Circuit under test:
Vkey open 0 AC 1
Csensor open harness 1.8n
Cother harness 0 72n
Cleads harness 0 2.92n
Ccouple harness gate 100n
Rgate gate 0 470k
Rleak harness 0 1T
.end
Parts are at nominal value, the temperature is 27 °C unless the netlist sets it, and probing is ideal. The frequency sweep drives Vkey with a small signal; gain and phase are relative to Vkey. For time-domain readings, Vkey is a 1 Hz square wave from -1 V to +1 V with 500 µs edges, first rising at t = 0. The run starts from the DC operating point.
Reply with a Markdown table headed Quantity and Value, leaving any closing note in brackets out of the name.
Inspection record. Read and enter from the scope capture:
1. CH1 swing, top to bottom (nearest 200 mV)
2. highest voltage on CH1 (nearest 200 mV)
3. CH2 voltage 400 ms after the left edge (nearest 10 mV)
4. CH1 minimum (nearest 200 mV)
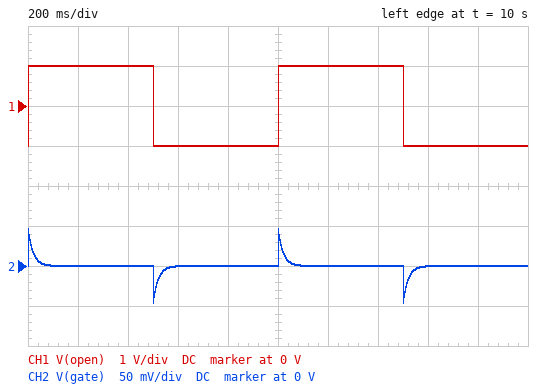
| Quantity | Value |
|---|---|
| CH1 swing, top to bottom | 2.0 V |
| highest voltage on CH1 | 1.0 V |
| CH2 voltage 400 ms after the left edge | 0 V |
| CH1 minimum | -1.0 V |
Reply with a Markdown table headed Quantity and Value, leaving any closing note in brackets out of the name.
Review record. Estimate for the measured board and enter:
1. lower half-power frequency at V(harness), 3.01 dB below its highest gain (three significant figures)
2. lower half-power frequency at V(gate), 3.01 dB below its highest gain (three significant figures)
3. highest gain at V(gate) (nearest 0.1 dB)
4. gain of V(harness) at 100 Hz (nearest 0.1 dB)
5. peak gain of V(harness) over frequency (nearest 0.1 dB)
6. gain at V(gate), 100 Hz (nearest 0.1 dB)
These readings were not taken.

| Quantity | Value |
|---|---|
| lower half-power frequency at V(harness), 3.01 dB below its highest gain | 6.16 Hz |
| lower half-power frequency at V(gate), 3.01 dB below its highest gain | 7.80 Hz |
| highest gain at V(gate) | -32.6 dB |
| gain of V(harness) at 100 Hz | -32.6 dB |
| peak gain of V(harness) over frequency | -32.6 dB |
| gain at V(gate), 100 Hz | -32.6 dB |
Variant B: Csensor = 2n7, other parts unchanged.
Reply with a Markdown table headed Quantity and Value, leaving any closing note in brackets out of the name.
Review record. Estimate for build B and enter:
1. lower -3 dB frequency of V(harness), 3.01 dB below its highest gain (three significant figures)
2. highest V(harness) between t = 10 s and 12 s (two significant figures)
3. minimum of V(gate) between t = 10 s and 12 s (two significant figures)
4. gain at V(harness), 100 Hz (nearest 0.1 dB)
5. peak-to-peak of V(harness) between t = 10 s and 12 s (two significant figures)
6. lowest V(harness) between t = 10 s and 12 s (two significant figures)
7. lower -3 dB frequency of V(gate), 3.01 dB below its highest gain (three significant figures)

| Quantity | Value |
|---|---|
| lower -3 dB frequency of V(harness), 3.01 dB below its highest gain | 6.09 Hz |
| highest V(harness) between t = 10 s and 12 s | 69 mV |
| minimum of V(gate) between t = 10 s and 12 s | -69 mV |
| gain at V(harness), 100 Hz | -29.2 dB |
| peak-to-peak of V(harness) between t = 10 s and 12 s | 110 mV |
| lowest V(harness) between t = 10 s and 12 s | -39 mV |
| lower -3 dB frequency of V(gate), 3.01 dB below its highest gain | 7.75 Hz |
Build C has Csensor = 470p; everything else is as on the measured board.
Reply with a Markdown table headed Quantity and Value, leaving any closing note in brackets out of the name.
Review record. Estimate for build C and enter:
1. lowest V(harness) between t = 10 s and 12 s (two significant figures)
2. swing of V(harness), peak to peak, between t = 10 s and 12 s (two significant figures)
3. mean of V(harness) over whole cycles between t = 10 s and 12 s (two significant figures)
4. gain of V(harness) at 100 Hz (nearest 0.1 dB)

| Quantity | Value |
|---|---|
| lowest V(harness) between t = 10 s and 12 s | -7.0 mV |
| swing of V(harness), peak to peak, between t = 10 s and 12 s | 19 mV |
| mean of V(harness) over whole cycles between t = 10 s and 12 s | 2.7 mV |
| gain of V(harness) at 100 Hz | -44.1 dB |
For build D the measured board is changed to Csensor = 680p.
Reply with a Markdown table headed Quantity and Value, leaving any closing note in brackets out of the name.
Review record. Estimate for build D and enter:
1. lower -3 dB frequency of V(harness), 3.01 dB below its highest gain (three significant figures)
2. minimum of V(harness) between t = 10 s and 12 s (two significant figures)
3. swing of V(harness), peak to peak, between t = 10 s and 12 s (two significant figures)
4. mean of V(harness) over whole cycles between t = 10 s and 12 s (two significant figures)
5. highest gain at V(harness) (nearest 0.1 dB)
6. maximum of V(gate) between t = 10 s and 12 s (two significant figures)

| Quantity | Value |
|---|---|
| lower -3 dB frequency of V(harness), 3.01 dB below its highest gain | 6.24 Hz |
| minimum of V(harness) between t = 10 s and 12 s | -10 mV |
| swing of V(harness), peak to peak, between t = 10 s and 12 s | 28 mV |
| mean of V(harness) over whole cycles between t = 10 s and 12 s | 3.9 mV |
| highest gain at V(harness) | -40.9 dB |
| maximum of V(gate) between t = 10 s and 12 s | 18 mV |
